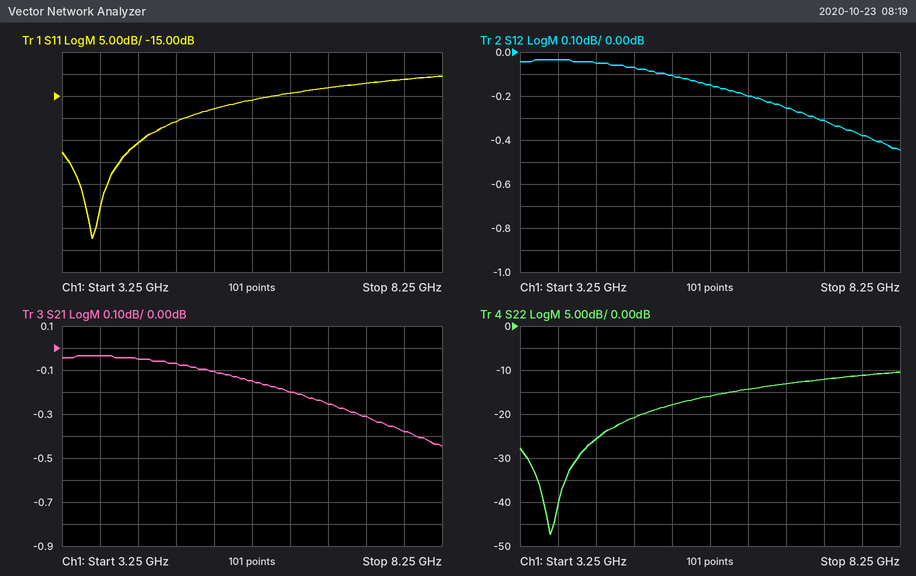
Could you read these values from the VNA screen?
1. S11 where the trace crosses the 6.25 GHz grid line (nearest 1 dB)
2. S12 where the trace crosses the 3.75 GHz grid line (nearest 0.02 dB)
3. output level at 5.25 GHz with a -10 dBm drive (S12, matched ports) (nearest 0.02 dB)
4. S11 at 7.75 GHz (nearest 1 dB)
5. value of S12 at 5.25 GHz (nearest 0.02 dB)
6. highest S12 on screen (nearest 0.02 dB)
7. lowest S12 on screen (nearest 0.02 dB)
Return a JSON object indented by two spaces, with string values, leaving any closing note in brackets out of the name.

{
  "S11 where the trace crosses the 6.25 GHz grid line": "-14 dB",
  "S12 where the trace crosses the 3.75 GHz grid line": "-0.04 dB",
  "output level at 5.25 GHz with a -10 dBm drive (S12, matched ports)": "-10.10 dBm",
  "S11 at 7.75 GHz": "-11 dB",
  "value of S12 at 5.25 GHz": "-0.10 dB",
  "highest S12 on screen": "-0.04 dB",
  "lowest S12 on screen": "-0.44 dB"
}
